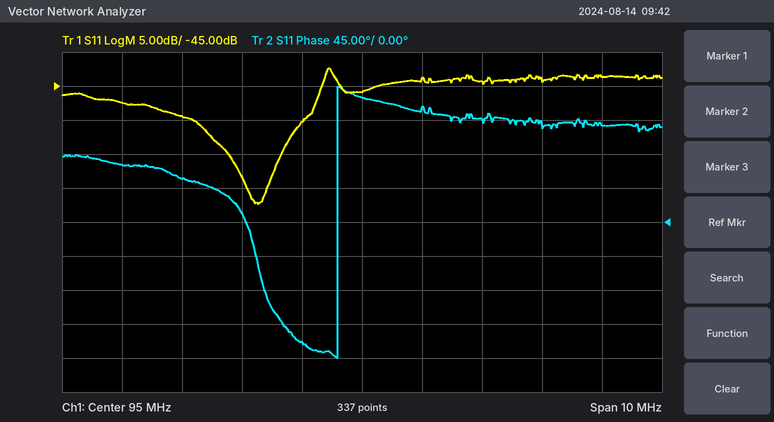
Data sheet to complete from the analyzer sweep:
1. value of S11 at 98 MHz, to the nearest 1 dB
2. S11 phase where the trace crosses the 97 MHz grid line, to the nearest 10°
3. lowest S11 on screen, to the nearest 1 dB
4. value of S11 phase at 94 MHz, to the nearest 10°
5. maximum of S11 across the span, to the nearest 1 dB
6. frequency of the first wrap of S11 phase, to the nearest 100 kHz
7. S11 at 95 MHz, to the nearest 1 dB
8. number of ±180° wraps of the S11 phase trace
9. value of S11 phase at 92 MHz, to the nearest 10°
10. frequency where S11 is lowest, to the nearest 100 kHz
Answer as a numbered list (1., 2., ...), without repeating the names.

1. -44 dB
2. 140°
3. -62 dB
4. -160°
5. -42 dB
6. 94.6 MHz
7. -46 dB
8. 1
9. 60°
10. 93.3 MHz
